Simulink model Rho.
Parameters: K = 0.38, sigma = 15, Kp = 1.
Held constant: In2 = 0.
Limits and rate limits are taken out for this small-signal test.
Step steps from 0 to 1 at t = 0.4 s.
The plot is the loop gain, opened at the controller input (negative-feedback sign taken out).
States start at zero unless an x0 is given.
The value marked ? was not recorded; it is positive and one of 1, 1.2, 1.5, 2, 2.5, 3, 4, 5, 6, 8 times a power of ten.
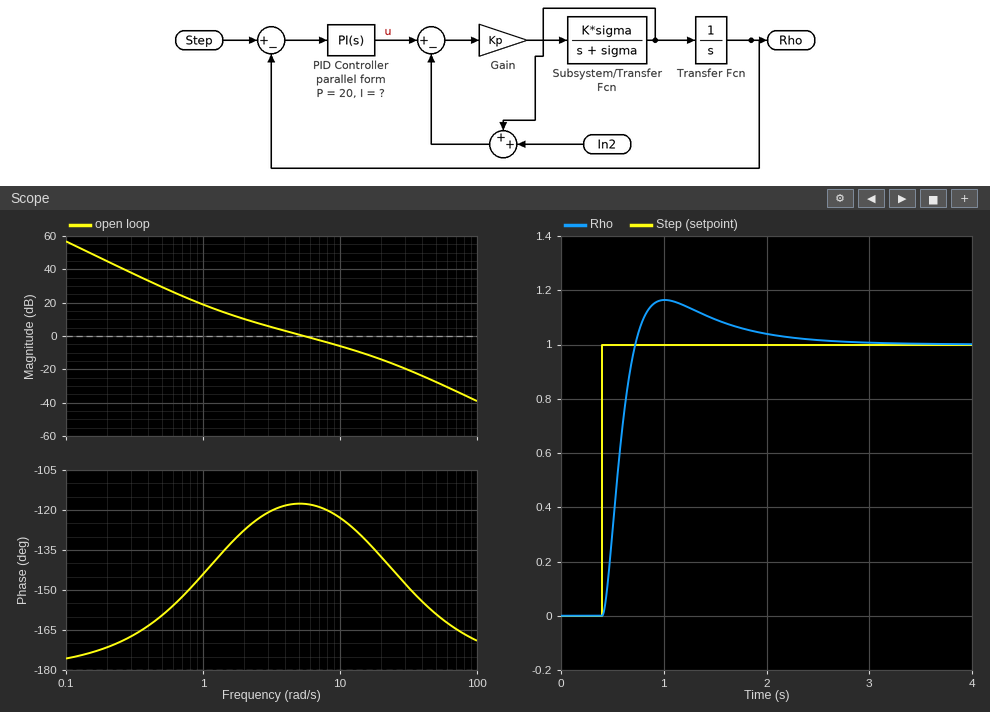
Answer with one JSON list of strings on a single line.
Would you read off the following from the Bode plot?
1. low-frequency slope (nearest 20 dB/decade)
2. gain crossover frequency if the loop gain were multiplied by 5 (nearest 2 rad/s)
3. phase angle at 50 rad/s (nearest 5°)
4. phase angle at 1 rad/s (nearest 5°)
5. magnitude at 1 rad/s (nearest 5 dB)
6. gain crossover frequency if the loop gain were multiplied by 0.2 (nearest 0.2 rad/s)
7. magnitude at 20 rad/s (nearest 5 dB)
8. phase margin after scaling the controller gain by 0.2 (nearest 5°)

["-40 dB/decade", "20 rad/s", "-160°", "-145°", "20 dB", "1.4 rad/s", "-15 dB", "45°"]
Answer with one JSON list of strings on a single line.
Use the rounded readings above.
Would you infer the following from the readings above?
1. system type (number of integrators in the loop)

["2"]
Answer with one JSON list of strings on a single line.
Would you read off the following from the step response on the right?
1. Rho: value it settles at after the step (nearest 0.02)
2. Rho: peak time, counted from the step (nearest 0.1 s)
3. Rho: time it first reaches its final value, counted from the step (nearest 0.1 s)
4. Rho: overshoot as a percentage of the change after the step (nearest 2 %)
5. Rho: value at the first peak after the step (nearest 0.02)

["1.00", "0.6 s", "0.3 s", "16 %", "1.16"]
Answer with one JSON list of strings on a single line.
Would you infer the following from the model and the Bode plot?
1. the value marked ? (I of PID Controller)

["25"]
